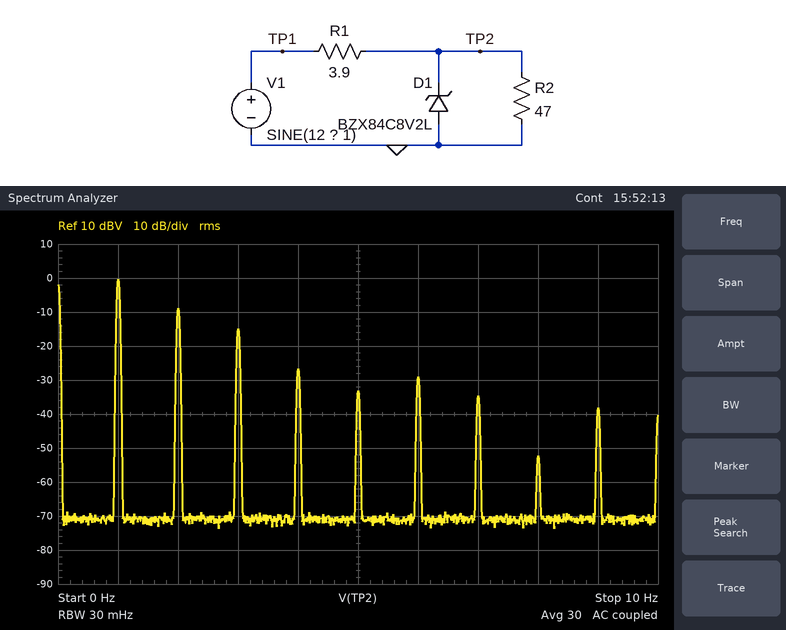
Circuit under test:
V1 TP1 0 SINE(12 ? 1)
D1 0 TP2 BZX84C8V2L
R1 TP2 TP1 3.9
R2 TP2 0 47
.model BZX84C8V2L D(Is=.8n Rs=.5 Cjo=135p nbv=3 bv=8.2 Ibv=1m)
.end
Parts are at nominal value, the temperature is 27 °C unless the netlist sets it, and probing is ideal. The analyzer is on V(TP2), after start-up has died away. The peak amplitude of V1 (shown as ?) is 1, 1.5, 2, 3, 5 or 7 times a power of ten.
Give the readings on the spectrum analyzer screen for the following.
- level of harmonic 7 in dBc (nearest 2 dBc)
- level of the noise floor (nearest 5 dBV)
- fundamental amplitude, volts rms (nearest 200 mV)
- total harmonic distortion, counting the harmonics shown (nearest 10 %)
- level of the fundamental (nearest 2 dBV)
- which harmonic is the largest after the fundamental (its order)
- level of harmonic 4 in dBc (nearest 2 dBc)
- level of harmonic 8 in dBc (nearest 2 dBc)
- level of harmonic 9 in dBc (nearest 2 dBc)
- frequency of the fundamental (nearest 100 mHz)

-34 dBc
-70 dBV
1.0 V
40 %
0 dBV
2
-26 dBc
-52 dBc
-38 dBc
1.0 Hz
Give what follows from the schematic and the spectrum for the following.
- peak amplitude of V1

5 V
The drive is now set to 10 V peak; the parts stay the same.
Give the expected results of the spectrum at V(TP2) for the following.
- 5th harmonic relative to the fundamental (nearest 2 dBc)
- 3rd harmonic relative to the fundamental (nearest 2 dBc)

-26 dBc
-20 dBc
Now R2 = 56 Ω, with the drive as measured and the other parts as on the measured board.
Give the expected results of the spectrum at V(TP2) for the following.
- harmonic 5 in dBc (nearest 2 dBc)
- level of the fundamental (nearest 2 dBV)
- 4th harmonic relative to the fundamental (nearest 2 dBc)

-36 dBc
0 dBV
-24 dBc
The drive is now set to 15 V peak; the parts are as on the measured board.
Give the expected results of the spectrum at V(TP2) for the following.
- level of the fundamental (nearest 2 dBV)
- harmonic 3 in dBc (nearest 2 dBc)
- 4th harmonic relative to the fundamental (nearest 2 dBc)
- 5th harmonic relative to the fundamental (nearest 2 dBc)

12 dBV
-40 dBc
-20 dBc
-24 dBc
